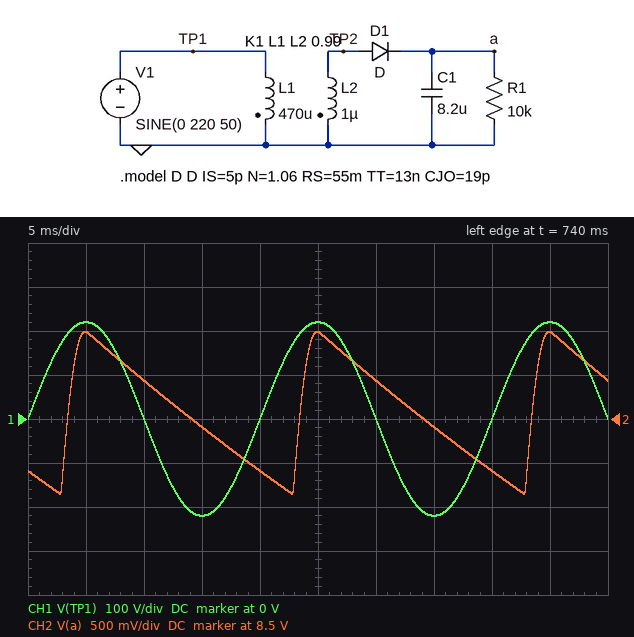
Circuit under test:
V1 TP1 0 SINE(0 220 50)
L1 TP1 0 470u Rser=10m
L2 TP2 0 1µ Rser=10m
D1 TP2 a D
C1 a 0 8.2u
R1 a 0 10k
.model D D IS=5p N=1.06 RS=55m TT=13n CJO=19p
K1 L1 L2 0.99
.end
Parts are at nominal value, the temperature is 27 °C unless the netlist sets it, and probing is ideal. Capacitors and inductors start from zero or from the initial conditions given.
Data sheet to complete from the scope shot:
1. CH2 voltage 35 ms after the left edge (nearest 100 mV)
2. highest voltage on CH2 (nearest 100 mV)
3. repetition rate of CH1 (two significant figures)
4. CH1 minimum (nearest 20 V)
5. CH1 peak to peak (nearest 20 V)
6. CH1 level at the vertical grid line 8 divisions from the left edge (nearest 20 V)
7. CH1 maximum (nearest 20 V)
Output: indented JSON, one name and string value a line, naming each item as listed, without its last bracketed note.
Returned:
{
  "CH2 voltage 35 ms after the left edge": "8.4 V",
  "highest voltage on CH2": "9.5 V",
  "repetition rate of CH1": "50 Hz",
  "CH1 minimum": "-220 V",
  "CH1 peak to peak": "440 V",
  "CH1 level at the vertical grid line 8 divisions from the left edge": "0 V",
  "CH1 maximum": "220 V"
}
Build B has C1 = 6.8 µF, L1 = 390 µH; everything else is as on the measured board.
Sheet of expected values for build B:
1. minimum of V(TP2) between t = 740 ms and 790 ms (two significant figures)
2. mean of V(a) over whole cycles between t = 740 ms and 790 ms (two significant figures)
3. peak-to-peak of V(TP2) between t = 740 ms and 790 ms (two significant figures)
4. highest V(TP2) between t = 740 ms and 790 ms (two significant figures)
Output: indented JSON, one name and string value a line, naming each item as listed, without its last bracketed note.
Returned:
{
  "minimum of V(TP2) between t = 740 ms and 790 ms": "-11 V",
  "mean of V(a) over whole cycles between t = 740 ms and 790 ms": "9.3 V",
  "peak-to-peak of V(TP2) between t = 740 ms and 790 ms": "22 V",
  "highest V(TP2) between t = 740 ms and 790 ms": "11 V"
}
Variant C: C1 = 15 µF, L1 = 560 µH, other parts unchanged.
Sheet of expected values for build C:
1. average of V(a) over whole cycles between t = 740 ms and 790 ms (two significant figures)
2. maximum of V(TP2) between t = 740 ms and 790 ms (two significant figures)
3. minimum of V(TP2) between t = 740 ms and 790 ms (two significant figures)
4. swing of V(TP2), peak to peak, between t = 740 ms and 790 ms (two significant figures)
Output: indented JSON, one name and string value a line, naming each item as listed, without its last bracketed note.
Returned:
{
  "average of V(a) over whole cycles between t = 740 ms and 790 ms": "8.2 V",
  "maximum of V(TP2) between t = 740 ms and 790 ms": "9.2 V",
  "minimum of V(TP2) between t = 740 ms and 790 ms": "-9.2 V",
  "swing of V(TP2), peak to peak, between t = 740 ms and 790 ms": "18 V"
}
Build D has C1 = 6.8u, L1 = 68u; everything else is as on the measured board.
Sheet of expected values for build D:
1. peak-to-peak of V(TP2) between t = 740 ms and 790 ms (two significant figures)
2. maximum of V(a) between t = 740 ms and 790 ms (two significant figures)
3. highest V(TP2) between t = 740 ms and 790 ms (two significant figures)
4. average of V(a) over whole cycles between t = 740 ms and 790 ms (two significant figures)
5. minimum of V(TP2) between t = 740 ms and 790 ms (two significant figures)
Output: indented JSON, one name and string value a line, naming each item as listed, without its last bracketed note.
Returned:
{
  "peak-to-peak of V(TP2) between t = 740 ms and 790 ms": "48 V",
  "maximum of V(a) between t = 740 ms and 790 ms": "23 V",
  "highest V(TP2) between t = 740 ms and 790 ms": "24 V",
  "average of V(a) over whole cycles between t = 740 ms and 790 ms": "21 V",
  "minimum of V(TP2) between t = 740 ms and 790 ms": "-24 V"
}
